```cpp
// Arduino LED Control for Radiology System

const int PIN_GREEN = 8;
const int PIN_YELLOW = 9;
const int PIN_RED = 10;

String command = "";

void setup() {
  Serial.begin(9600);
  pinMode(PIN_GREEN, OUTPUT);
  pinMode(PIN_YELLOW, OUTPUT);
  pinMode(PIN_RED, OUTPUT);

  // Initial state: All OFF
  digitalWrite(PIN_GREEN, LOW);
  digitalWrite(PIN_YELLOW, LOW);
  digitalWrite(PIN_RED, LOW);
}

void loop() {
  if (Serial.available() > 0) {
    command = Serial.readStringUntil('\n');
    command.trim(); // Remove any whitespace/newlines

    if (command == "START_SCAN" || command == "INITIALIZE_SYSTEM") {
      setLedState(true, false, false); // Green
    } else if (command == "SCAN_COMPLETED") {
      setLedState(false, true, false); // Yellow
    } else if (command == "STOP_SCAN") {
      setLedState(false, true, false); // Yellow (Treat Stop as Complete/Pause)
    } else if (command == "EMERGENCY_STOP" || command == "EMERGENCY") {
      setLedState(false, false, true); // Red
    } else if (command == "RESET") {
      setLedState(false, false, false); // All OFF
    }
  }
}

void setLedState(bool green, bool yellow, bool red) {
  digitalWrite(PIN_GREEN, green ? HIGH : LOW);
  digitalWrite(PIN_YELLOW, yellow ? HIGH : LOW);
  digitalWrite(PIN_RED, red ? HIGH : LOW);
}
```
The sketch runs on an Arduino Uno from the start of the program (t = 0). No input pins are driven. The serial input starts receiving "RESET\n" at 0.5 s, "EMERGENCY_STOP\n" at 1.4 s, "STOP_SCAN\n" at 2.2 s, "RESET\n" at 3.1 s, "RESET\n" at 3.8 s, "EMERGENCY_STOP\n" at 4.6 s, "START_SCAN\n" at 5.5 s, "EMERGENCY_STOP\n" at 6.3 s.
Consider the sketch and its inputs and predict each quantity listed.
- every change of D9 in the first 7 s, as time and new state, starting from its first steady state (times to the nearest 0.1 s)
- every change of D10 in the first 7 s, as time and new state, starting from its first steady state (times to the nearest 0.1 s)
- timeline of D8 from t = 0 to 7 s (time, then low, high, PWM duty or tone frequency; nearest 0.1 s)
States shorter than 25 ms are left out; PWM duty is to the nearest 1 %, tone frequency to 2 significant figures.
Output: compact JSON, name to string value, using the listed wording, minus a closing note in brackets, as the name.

{"every change of D9 in the first 7 s, as time and new state, starting from its first steady state": "0 s low; 2.2 s high; 3.1 s low", "every change of D10 in the first 7 s, as time and new state, starting from its first steady state": "0 s low; 1.4 s high; 2.2 s low; 4.6 s high; 5.5 s low; 6.3 s high", "timeline of D8 from t = 0 to 7 s": "0 s low; 5.5 s high; 6.3 s low"}
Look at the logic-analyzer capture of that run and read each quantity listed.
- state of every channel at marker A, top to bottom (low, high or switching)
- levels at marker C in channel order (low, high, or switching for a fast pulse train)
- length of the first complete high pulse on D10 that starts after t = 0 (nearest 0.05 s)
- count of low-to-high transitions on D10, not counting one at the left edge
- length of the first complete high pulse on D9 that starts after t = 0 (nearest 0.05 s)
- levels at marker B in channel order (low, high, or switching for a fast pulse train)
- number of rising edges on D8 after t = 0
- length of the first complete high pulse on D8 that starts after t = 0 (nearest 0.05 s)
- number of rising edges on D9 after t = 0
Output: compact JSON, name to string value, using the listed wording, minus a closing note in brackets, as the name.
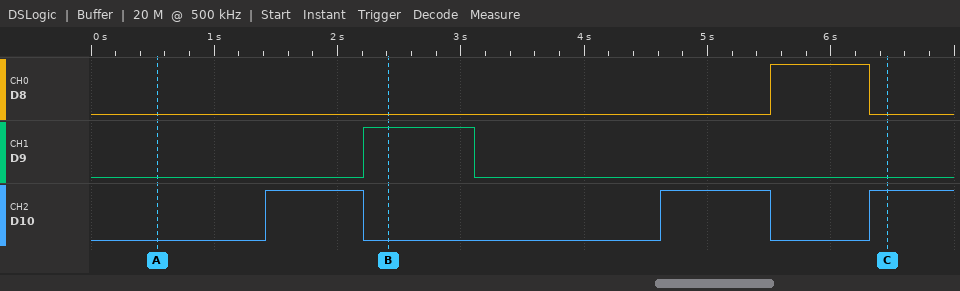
{"state of every channel at marker A, top to bottom": "D8 low, D9 low, D10 low", "levels at marker C in channel order": "D8 low, D9 low, D10 high", "length of the first complete high pulse on D10 that starts after t = 0": "0.80 s", "count of low-to-high transitions on D10, not counting one at the left edge": "3", "length of the first complete high pulse on D9 that starts after t = 0": "0.90 s", "levels at marker B in channel order": "D8 low, D9 high, D10 low", "number of rising edges on D8 after t = 0": "1", "length of the first complete high pulse on D8 that starts after t = 0": "0.80 s", "number of rising edges on D9 after t = 0": "1"}
